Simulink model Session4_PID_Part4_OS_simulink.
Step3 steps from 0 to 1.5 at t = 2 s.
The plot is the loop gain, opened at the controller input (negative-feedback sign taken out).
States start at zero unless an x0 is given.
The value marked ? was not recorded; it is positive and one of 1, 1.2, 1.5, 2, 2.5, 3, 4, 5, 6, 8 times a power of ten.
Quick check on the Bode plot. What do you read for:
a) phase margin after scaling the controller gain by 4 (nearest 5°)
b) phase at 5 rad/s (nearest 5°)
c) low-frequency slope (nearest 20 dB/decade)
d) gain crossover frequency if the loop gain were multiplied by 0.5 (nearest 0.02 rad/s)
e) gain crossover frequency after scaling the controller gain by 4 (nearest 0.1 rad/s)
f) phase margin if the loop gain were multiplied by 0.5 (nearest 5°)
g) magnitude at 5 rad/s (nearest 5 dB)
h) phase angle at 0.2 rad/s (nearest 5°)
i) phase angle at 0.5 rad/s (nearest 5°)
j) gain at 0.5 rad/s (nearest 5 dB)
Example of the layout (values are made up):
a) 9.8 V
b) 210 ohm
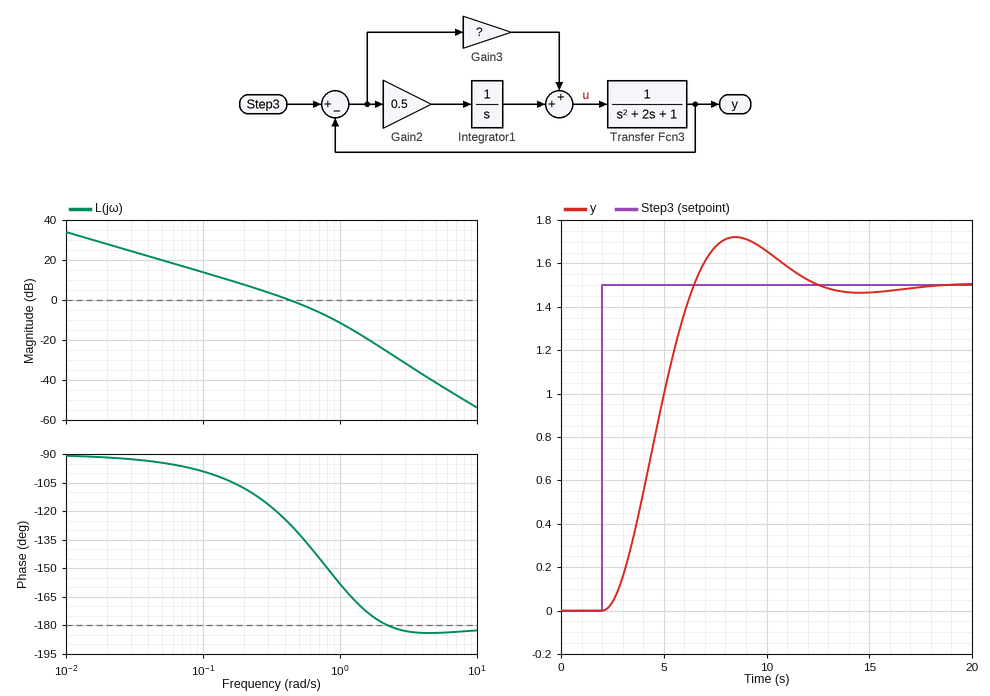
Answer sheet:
a) 20°
b) -185°
c) -20 dB/decade
d) 0.24 rad/s
e) 1.0 rad/s
f) 70°
g) -40 dB
h) -110°
i) -130°
j) 0 dB
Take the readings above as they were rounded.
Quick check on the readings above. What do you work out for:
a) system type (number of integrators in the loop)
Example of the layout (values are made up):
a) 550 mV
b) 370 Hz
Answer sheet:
a) 1
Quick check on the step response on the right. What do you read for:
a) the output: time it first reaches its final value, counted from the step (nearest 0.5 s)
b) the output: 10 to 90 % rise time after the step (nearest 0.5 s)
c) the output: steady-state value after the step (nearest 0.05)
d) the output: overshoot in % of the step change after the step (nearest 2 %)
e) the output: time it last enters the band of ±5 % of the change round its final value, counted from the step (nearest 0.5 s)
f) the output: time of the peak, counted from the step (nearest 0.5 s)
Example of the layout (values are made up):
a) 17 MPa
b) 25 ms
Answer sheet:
a) 4.5 s
b) 3.0 s
c) 1.50
d) 14 %
e) 9.0 s
f) 6.5 s
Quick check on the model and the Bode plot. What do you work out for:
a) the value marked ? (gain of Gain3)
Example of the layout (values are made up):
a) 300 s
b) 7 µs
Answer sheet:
a) 0.2
